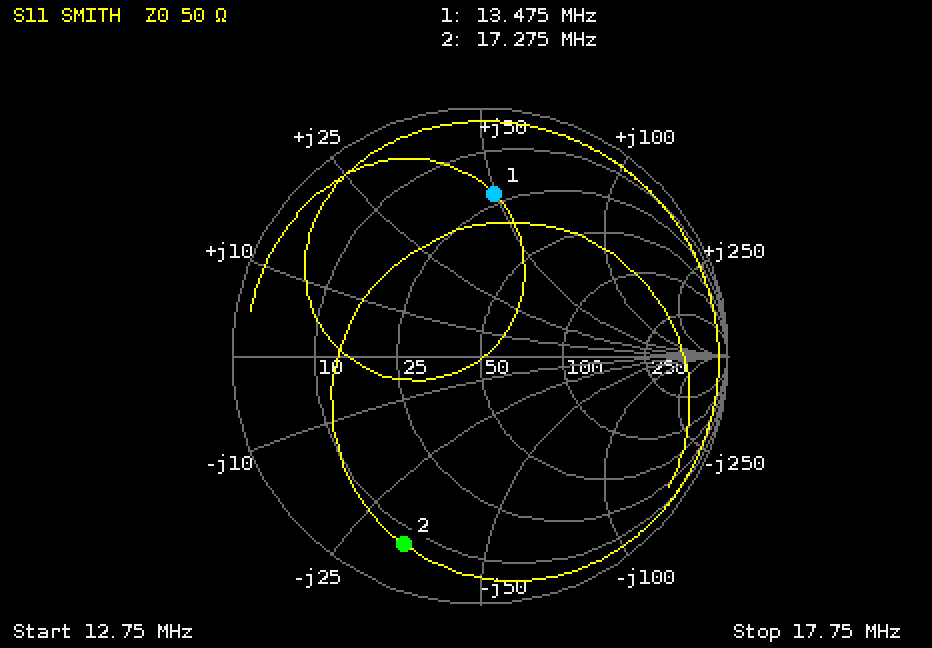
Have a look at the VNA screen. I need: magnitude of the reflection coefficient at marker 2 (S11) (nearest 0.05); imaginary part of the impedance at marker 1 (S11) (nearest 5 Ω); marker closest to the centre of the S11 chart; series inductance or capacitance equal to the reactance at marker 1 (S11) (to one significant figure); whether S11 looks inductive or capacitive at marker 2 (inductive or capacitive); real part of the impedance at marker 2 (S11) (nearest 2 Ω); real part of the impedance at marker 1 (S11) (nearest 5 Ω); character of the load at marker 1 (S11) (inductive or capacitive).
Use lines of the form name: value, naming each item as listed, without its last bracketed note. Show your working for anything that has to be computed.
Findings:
magnitude of the reflection coefficient at marker 2 (S11): 0.80
imaginary part of the impedance at marker 1 (S11): +50 Ω
marker closest to the centre of the S11 chart: marker 1
series inductance or capacitance equal to the reactance at marker 1 (S11): L = 50 Ω/(2π × 13.475 MHz) ≈ 591 nH, so 600 nH to one significant figure
whether S11 looks inductive or capacitive at marker 2: capacitive
real part of the impedance at marker 2 (S11): 8 Ω
real part of the impedance at marker 1 (S11): 20 Ω
character of the load at marker 1 (S11): inductive
